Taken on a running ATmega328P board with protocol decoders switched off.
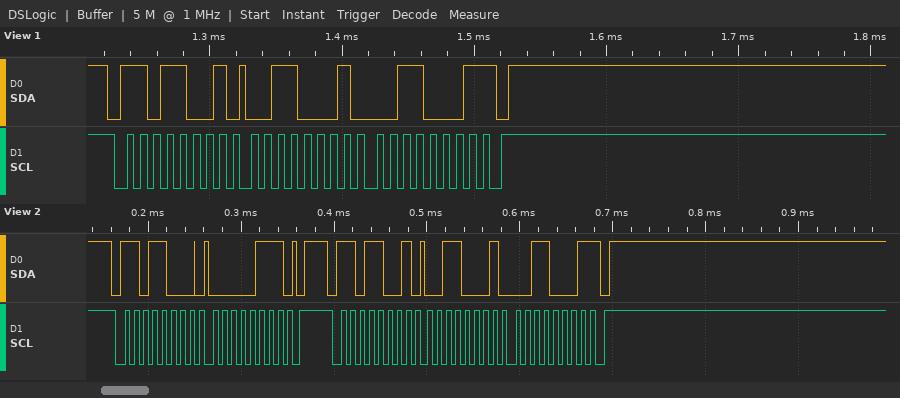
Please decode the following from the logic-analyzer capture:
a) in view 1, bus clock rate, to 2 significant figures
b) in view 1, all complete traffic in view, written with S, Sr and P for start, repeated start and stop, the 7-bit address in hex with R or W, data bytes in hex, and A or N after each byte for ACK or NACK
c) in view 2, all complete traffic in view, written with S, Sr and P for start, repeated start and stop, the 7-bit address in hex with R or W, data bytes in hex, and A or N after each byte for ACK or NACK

100 kHz
S 6CR A 31 A 31 N P
S 6CW A 07 A P S 6CR A 31 A 31 N P
